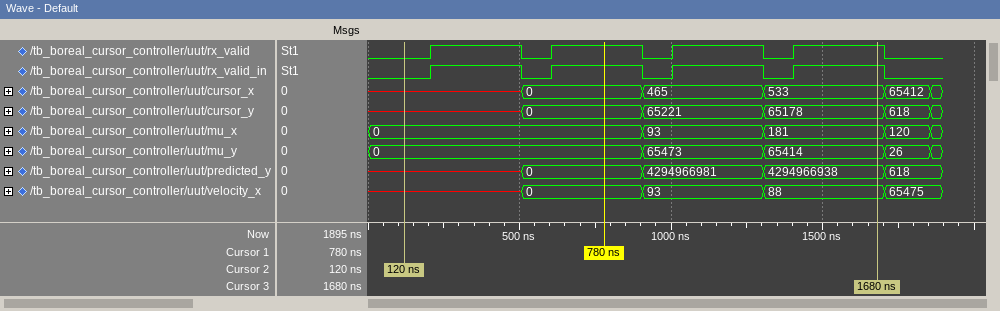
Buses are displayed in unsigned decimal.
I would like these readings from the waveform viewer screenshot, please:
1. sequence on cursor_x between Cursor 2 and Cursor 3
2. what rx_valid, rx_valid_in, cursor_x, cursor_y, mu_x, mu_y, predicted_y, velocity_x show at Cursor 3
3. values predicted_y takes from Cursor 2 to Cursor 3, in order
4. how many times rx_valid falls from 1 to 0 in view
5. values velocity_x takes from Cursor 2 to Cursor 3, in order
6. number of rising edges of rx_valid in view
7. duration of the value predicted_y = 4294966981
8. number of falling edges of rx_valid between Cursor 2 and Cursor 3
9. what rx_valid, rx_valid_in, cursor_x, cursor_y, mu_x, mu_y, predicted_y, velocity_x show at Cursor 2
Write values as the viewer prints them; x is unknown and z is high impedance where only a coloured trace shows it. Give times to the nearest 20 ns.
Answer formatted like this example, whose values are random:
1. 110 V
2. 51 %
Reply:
1. x, 0, 465, 533
2. rx_valid=1, rx_valid_in=1, cursor_x=533, cursor_y=65178, mu_x=181, mu_y=65414, predicted_y=4294966938, velocity_x=88
3. x, 0, 4294966981, 4294966938
4. 4
5. x, 0, 93, 88
6. 4
7. 400 ns
8. 3
9. rx_valid=0, rx_valid_in=0, cursor_x=x, cursor_y=x, mu_x=0, mu_y=0, predicted_y=x, velocity_x=x
